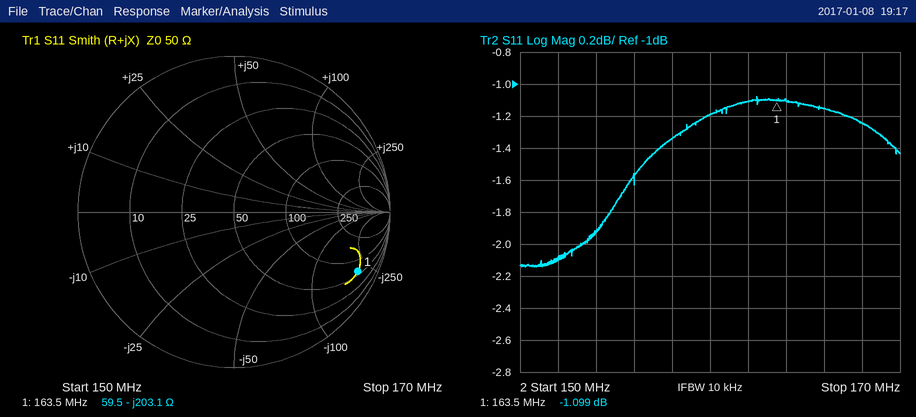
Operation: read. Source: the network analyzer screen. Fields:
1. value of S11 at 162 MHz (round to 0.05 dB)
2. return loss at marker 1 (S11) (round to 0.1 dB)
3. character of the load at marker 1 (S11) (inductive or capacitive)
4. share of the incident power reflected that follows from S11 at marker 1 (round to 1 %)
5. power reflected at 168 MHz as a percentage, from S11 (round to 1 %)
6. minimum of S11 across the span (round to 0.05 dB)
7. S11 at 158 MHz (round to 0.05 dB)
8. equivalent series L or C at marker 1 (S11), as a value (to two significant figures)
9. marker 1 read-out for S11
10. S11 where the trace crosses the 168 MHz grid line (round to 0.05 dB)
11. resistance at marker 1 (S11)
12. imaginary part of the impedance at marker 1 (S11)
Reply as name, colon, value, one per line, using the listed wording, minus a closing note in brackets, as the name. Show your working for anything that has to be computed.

value of S11 at 162 MHz: -1.10 dB
return loss at marker 1 (S11): 1.1 dB
character of the load at marker 1 (S11): capacitive
share of the incident power reflected that follows from S11 at marker 1: 10^(-1.099/10) ≈ 78 %
power reflected at 168 MHz as a percentage, from S11: 10^(-1.25/10) ≈ 75 %
minimum of S11 across the span: -2.15 dB
S11 at 158 MHz: -1.35 dB
equivalent series L or C at marker 1 (S11), as a value: C = 1/(2π × 163.5 MHz × 203.1 Ω) ≈ 4.8 pF
marker 1 read-out for S11: -1.099 dB
S11 where the trace crosses the 168 MHz grid line: -1.25 dB
resistance at marker 1: 59.5 Ω
imaginary part of the impedance at marker 1: -203.1 Ω
